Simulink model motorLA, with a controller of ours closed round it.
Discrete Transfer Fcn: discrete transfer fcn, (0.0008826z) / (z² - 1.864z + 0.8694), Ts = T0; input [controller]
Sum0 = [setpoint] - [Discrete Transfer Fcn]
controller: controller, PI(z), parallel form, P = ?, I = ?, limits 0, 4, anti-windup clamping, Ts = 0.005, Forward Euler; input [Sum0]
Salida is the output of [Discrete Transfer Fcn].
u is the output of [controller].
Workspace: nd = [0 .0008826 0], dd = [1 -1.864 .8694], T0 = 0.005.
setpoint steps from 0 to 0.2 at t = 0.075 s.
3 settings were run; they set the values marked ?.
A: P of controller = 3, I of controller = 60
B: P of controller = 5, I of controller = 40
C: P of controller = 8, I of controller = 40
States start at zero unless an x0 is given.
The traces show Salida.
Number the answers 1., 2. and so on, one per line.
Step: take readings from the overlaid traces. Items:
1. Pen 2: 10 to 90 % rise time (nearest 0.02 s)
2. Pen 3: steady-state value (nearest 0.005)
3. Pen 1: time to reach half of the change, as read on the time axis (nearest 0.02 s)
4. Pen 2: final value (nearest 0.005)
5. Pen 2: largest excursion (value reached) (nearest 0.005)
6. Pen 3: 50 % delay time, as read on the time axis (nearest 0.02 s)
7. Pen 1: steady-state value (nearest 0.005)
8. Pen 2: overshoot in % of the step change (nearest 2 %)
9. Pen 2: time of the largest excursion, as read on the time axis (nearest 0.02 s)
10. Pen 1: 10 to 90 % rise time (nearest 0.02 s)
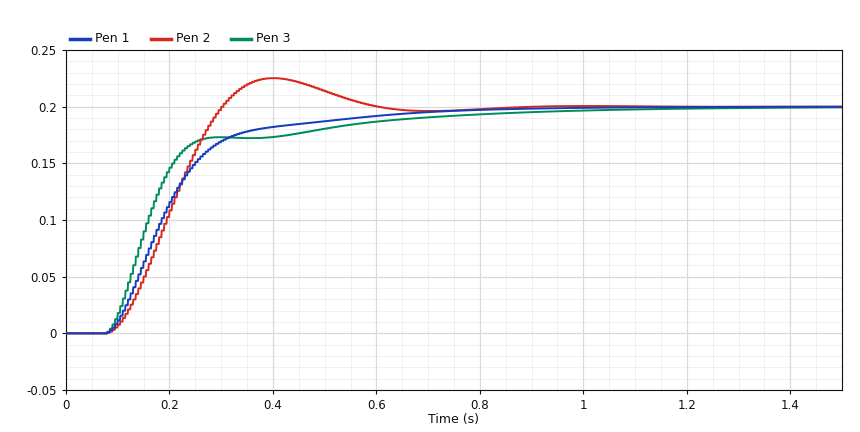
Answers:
1. 0.16 s
2. 0.200
3. 0.18 s
4. 0.200
5. 0.225
6. 0.16 s
7. 0.200
8. 12 %
9. 0.40 s
10. 0.26 s
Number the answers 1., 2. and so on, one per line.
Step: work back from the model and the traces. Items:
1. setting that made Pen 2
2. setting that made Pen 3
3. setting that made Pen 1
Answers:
1. A
2. C
3. B
